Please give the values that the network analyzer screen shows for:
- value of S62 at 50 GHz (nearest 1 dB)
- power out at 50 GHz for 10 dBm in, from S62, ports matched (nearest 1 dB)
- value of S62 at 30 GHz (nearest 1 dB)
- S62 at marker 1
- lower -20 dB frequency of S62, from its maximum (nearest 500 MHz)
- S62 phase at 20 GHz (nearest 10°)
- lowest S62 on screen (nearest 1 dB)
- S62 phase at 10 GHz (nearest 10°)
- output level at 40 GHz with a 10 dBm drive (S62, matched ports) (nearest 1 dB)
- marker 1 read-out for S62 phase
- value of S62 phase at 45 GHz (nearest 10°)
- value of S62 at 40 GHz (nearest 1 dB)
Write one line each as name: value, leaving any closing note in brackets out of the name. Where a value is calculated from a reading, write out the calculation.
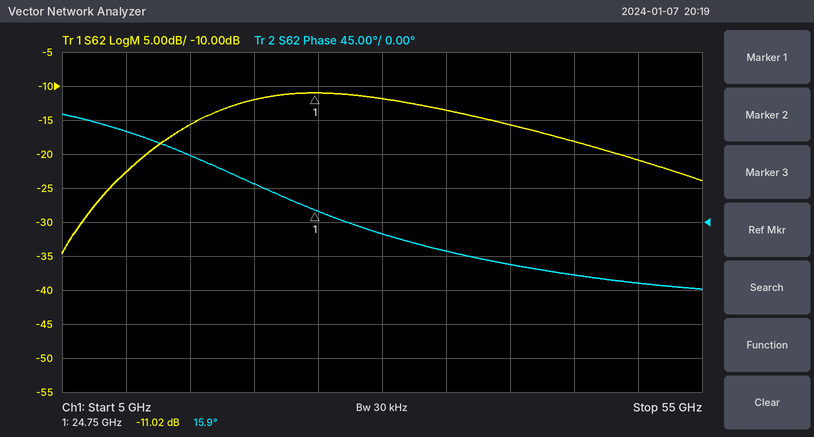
value of S62 at 50 GHz: -21 dB
power out at 50 GHz for 10 dBm in, from S62, ports matched: 10 dBm + (-21 dB) = -11 dBm
value of S62 at 30 GHz: -12 dB
S62 at marker 1: -11.02 dB
lower -20 dB frequency of S62, from its maximum: 6.0 GHz
S62 phase at 20 GHz: 50°
lowest S62 on screen: -35 dB
S62 phase at 10 GHz: 120°
output level at 40 GHz with a 10 dBm drive (S62, matched ports): 10 dBm + (-16 dB) = -6 dBm
marker 1 read-out for S62 phase: 15.9°
value of S62 phase at 45 GHz: -70°
value of S62 at 40 GHz: -16 dB
